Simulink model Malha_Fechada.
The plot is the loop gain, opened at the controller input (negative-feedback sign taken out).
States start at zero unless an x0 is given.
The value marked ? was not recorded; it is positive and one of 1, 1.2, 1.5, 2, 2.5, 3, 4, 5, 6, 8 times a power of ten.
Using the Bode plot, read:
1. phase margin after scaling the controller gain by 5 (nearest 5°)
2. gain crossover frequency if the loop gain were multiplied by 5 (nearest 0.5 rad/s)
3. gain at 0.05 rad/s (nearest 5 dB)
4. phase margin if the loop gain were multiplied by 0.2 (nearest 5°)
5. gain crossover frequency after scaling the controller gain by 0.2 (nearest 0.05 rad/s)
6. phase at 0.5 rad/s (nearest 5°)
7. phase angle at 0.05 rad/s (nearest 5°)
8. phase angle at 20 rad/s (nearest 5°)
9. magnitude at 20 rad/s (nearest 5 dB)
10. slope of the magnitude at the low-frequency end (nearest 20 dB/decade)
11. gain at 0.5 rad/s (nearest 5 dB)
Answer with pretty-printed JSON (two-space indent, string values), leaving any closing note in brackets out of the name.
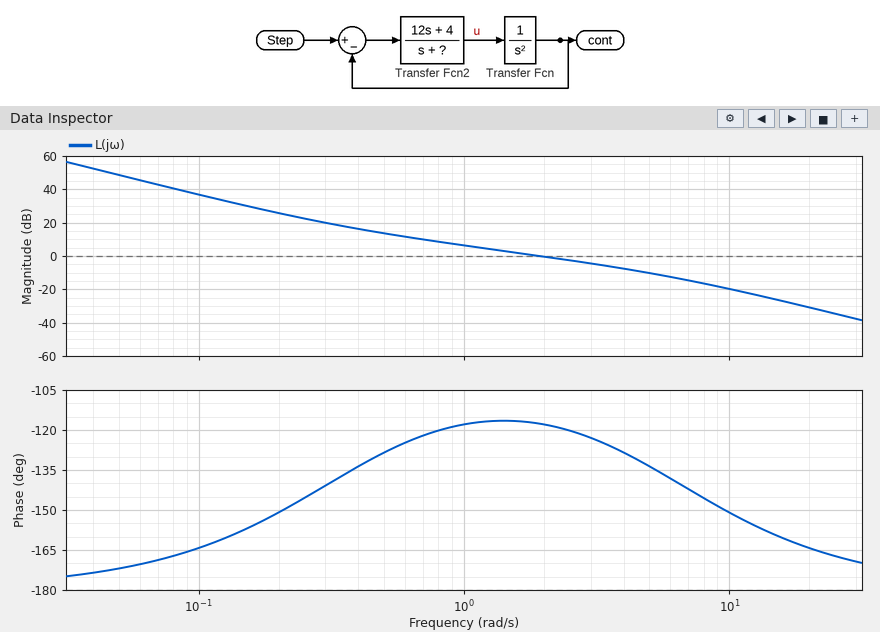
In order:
{
  "phase margin after scaling the controller gain by 5": "40°",
  "gain crossover frequency if the loop gain were multiplied by 5": "6.5 rad/s",
  "gain at 0.05 rad/s": "50 dB",
  "phase margin if the loop gain were multiplied by 0.2": "50°",
  "gain crossover frequency after scaling the controller gain by 0.2": "0.50 rad/s",
  "phase at 0.5 rad/s": "-130°",
  "phase angle at 0.05 rad/s": "-170°",
  "phase angle at 20 rad/s": "-165°",
  "magnitude at 20 rad/s": "-30 dB",
  "slope of the magnitude at the low-frequency end": "-40 dB/decade",
  "gain at 0.5 rad/s": "15 dB"
}
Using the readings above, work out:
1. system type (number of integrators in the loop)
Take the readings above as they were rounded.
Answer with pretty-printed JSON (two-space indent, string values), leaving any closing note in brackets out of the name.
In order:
{
  "system type": "2"
}
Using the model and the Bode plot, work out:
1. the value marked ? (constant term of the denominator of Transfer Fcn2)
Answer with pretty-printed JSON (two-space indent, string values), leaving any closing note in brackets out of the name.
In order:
{
  "the value marked ?": "6"
}
